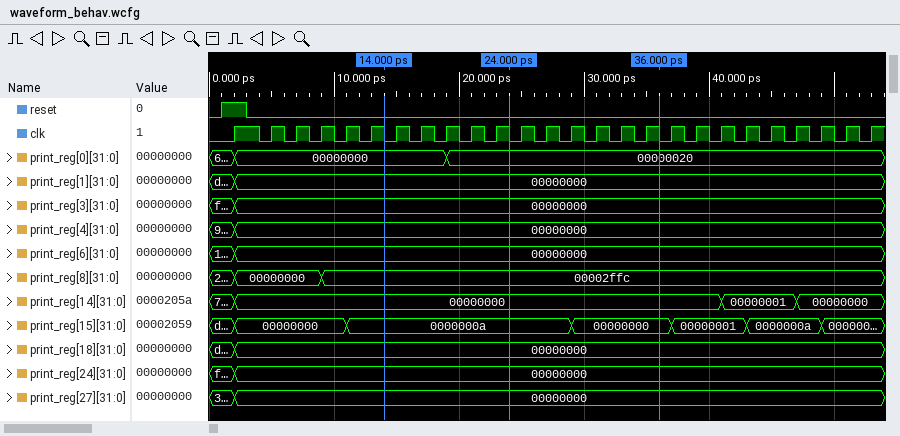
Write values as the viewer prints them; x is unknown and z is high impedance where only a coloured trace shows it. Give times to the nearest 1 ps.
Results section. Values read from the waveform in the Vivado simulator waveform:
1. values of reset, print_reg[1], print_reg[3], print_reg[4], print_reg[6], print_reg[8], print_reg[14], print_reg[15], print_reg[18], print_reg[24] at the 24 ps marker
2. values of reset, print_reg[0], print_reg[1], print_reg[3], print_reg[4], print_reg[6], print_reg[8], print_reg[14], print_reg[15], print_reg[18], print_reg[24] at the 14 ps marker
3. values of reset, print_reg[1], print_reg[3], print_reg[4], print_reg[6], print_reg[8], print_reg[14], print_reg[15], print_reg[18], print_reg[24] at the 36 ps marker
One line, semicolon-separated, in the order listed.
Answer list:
reset=0, print_reg[1]=00000000, print_reg[3]=00000000, print_reg[4]=00000000, print_reg[6]=00000000, print_reg[8]=00002ffc, print_reg[14]=00000000, print_reg[15]=0000000a, print_reg[18]=00000000, print_reg[24]=00000000; reset=0, print_reg[0]=00000000, print_reg[1]=00000000, print_reg[3]=00000000, print_reg[4]=00000000, print_reg[6]=00000000, print_reg[8]=00002ffc, print_reg[14]=00000000, print_reg[15]=0000000a, print_reg[18]=00000000, print_reg[24]=00000000; reset=0, print_reg[1]=00000000, print_reg[3]=00000000, print_reg[4]=00000000, print_reg[6]=00000000, print_reg[8]=00002ffc, print_reg[14]=00000000, print_reg[15]=00000000, print_reg[18]=00000000, print_reg[24]=00000000
